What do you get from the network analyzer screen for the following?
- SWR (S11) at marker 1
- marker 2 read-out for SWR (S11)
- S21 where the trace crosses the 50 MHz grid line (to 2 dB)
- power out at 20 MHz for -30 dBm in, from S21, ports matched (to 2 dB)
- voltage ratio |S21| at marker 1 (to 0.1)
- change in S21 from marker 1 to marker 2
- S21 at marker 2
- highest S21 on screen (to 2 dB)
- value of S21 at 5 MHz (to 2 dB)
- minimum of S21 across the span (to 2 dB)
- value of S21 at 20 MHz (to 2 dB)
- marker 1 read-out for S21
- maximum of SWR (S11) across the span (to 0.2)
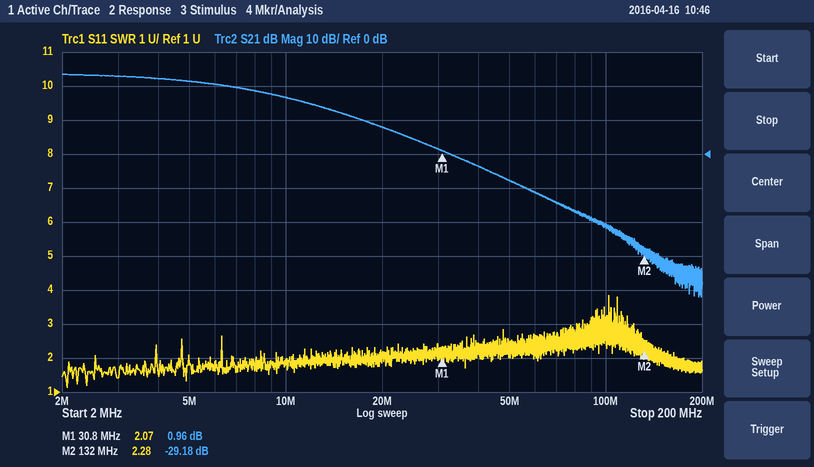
2.07
2.28
-8 dB
-22 dBm
1.1
-30.14 dB
-29.18 dB
24 dB
22 dB
-42 dB
8 dB
0.96 dB
3.8
